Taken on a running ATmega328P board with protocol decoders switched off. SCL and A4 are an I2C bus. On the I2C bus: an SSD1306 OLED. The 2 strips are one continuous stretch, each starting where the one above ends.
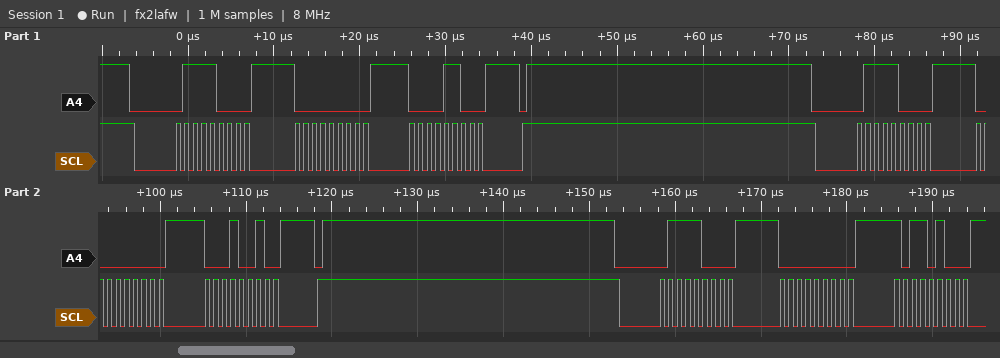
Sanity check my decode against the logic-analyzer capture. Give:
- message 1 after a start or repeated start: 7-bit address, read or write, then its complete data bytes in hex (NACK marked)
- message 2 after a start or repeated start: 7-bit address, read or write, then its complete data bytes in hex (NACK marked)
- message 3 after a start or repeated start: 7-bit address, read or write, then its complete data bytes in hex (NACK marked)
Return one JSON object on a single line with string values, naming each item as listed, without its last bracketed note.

{"message 1 after a start or repeated start: 7-bit address, read or write, then its complete data bytes in hex": "0x3C write: 00 0C", "message 2 after a start or repeated start: 7-bit address, read or write, then its complete data bytes in hex": "0x3C write: 00 12", "message 3 after a start or repeated start: 7-bit address, read or write, then its complete data bytes in hex": "0x3C write: 00 B4"}
